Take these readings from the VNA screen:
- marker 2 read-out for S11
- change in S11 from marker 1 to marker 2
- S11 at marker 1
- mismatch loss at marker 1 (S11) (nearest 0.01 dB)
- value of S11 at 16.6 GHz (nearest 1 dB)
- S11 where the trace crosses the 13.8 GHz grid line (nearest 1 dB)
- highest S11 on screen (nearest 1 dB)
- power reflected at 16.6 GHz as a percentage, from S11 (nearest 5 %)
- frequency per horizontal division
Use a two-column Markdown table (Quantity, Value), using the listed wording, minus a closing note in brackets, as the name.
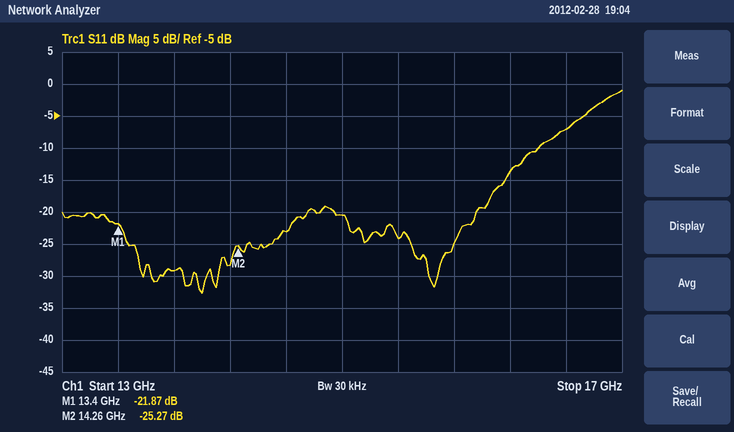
| Quantity | Value |
|---|---|
| marker 2 read-out for S11 | -25.27 dB |
| change in S11 from marker 1 to marker 2 | -3.40 dB |
| S11 at marker 1 | -21.87 dB |
| mismatch loss at marker 1 (S11) | 0.03 dB |
| value of S11 at 16.6 GHz | -7 dB |
| S11 where the trace crosses the 13.8 GHz grid line | -29 dB |
| highest S11 on screen | -1 dB |
| power reflected at 16.6 GHz as a percentage, from S11 | 20 % |
| frequency per horizontal division | 400 MHz |
